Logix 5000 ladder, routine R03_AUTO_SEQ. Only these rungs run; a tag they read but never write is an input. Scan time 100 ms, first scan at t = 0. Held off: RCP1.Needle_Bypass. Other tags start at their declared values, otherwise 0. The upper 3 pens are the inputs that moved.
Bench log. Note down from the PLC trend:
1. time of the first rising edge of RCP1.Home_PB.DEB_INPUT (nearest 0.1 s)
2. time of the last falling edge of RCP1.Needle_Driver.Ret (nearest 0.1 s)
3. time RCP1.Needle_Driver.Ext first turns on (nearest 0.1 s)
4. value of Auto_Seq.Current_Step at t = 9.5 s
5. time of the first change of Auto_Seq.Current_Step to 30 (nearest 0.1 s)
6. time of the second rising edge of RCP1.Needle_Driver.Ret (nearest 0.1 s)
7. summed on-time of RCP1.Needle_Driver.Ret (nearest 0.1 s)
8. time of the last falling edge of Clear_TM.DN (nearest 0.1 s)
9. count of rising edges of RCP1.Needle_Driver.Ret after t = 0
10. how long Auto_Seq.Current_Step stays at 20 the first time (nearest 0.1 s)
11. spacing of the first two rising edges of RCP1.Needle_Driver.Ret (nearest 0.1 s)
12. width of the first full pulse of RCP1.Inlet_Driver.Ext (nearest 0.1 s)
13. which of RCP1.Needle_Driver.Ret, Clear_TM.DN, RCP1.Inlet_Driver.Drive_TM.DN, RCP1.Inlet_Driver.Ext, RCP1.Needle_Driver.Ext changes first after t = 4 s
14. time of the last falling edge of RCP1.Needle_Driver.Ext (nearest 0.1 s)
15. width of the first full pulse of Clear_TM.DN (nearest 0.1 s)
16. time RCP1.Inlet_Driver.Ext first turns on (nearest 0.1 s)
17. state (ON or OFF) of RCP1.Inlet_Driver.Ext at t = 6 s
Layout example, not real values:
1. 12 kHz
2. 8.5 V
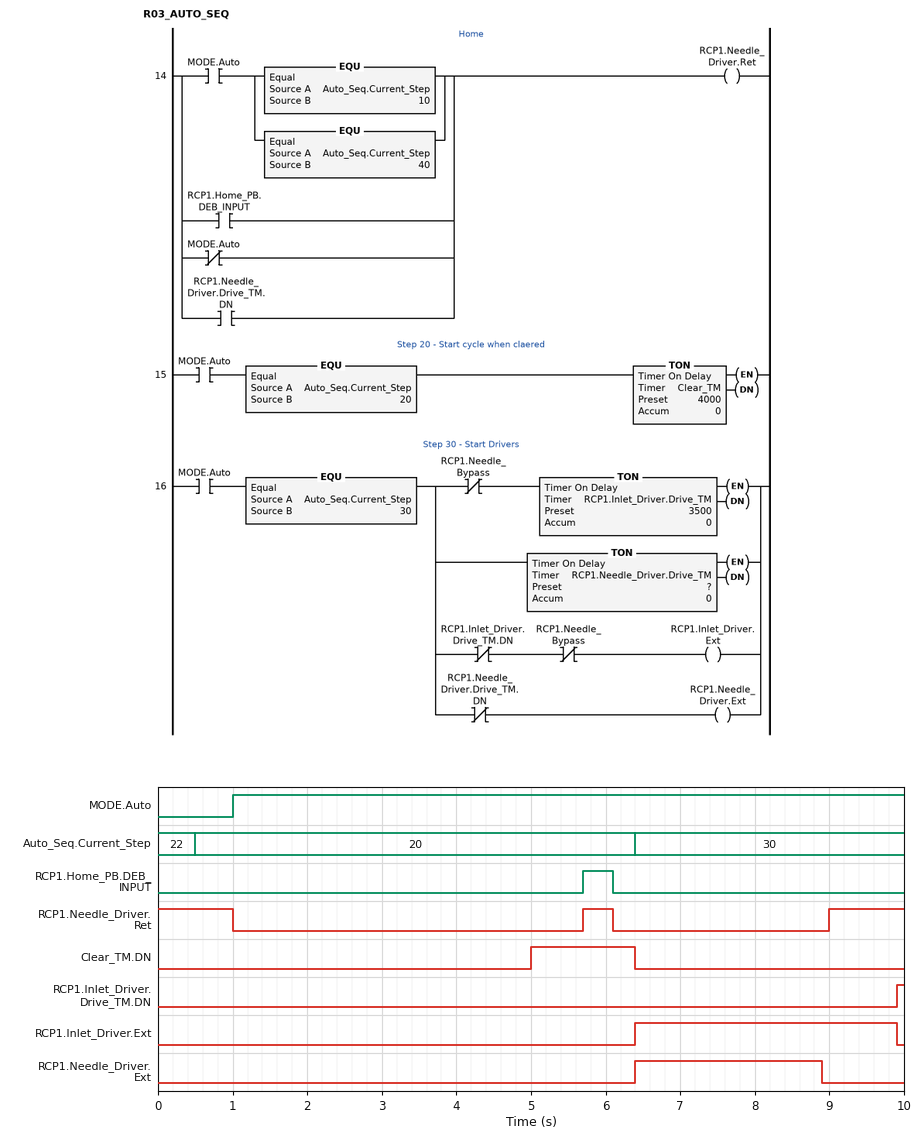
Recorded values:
1. 5.7 s
2. 6.1 s
3. 6.4 s
4. 30
5. 6.4 s
6. 9.0 s
7. 2.4 s
8. 6.4 s
9. 2
10. 5.9 s
11. 3.3 s
12. 3.5 s
13. Clear_TM.DN
14. 8.9 s
15. 1.4 s
16. 6.4 s
17. OFF
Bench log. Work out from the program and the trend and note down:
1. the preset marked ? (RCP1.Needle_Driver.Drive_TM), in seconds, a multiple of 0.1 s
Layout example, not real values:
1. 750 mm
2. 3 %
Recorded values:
1. 2.5 s
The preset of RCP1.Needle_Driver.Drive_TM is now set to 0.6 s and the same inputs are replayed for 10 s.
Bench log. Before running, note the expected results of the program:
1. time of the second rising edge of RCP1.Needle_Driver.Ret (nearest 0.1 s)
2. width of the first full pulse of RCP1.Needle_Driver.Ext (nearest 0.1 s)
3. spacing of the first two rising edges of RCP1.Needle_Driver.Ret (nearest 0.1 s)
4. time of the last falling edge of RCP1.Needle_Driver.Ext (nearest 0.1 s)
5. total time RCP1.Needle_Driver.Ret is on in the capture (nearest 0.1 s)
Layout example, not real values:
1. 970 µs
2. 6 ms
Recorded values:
1. 7.1 s
2. 0.6 s
3. 1.4 s
4. 7.0 s
5. 4.3 s
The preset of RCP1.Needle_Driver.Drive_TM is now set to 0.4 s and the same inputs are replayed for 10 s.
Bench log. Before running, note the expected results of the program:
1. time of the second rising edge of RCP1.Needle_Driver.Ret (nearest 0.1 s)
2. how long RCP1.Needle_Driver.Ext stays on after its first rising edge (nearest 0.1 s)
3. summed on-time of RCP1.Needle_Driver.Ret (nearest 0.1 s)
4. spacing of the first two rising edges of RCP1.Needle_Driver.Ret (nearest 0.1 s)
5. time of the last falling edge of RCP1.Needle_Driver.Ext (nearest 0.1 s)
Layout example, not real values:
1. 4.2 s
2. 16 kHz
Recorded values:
1. 6.9 s
2. 0.4 s
3. 4.5 s
4. 1.2 s
5. 6.8 s
